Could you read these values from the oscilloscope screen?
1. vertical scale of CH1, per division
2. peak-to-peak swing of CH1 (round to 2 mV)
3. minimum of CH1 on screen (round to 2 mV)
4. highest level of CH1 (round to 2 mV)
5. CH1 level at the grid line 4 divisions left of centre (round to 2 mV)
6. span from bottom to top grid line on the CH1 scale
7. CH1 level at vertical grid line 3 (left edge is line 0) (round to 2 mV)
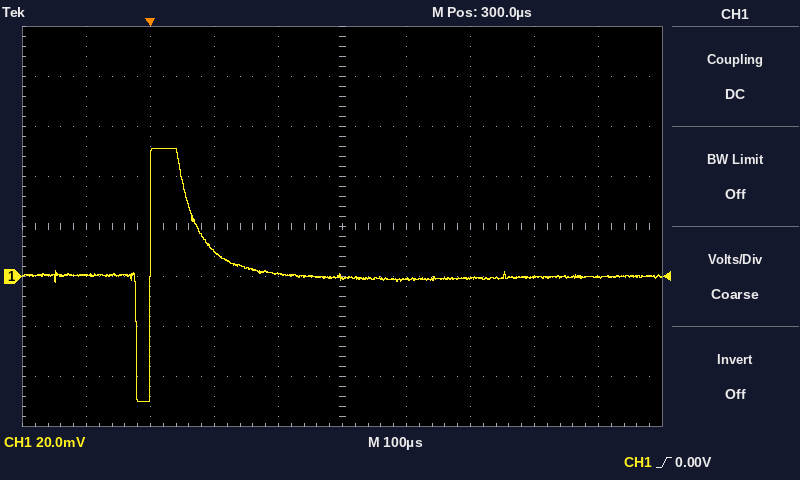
20 mV
102 mV
-50 mV
52 mV
0 mV
160 mV
10 mV
